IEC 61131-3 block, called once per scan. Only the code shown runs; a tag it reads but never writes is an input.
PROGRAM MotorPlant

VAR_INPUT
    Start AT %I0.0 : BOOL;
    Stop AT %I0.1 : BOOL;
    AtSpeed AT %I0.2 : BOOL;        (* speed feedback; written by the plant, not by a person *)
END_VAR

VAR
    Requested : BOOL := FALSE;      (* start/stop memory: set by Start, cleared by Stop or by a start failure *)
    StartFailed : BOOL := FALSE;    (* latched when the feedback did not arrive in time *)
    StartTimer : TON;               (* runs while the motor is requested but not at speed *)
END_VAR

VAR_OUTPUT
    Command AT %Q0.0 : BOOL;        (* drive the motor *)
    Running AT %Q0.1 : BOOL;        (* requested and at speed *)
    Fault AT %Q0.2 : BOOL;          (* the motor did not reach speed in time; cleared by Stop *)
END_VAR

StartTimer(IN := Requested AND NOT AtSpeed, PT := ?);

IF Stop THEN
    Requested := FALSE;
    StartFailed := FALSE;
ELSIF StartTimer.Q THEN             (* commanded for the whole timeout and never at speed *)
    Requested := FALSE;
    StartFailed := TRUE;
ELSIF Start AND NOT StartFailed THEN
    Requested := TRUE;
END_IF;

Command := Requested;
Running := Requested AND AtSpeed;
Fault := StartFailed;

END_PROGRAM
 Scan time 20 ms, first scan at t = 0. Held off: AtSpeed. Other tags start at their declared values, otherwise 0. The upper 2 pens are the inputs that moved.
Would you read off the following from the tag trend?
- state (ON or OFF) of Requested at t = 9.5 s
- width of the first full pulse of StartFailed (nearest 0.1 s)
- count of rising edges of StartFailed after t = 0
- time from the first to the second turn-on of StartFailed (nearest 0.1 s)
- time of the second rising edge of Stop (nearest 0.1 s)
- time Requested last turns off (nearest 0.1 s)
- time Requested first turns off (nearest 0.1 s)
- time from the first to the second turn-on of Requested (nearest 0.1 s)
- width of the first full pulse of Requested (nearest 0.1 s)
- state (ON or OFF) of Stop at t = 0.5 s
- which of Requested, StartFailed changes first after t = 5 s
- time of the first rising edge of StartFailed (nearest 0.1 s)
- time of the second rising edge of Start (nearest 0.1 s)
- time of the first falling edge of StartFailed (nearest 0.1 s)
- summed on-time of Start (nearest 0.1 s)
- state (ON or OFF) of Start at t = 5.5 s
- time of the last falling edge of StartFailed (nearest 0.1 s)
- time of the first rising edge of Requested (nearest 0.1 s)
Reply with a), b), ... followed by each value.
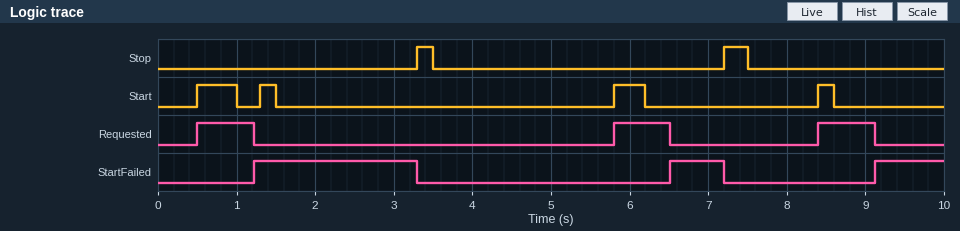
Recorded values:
a) OFF
b) 2.1 s
c) 3
d) 5.3 s
e) 7.2 s
f) 9.1 s
g) 1.2 s
h) 5.3 s
i) 0.7 s
j) OFF
k) Requested
l) 1.2 s
m) 1.3 s
n) 3.3 s
o) 1.3 s
p) OFF
q) 7.2 s
r) 0.5 s
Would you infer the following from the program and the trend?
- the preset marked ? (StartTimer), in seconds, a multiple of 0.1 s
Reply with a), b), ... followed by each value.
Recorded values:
a) 0.7 s
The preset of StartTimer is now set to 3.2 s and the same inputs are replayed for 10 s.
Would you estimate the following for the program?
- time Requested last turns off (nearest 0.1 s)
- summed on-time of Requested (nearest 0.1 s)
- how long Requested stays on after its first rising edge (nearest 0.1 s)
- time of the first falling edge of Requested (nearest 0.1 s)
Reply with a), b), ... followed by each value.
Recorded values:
a) 7.2 s
b) 5.8 s
c) 2.8 s
d) 3.3 s
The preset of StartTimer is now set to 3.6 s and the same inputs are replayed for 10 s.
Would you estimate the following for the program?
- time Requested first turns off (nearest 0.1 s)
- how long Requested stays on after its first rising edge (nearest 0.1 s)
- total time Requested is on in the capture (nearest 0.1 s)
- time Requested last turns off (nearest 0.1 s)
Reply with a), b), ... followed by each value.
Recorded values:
a) 3.3 s
b) 2.8 s
c) 5.8 s
d) 7.2 s
